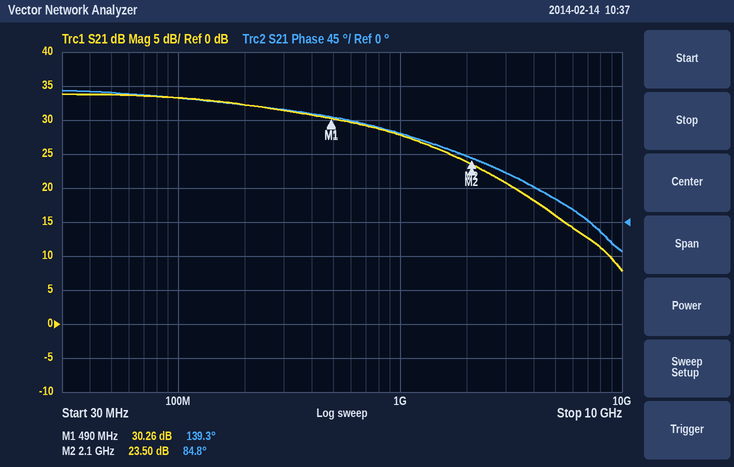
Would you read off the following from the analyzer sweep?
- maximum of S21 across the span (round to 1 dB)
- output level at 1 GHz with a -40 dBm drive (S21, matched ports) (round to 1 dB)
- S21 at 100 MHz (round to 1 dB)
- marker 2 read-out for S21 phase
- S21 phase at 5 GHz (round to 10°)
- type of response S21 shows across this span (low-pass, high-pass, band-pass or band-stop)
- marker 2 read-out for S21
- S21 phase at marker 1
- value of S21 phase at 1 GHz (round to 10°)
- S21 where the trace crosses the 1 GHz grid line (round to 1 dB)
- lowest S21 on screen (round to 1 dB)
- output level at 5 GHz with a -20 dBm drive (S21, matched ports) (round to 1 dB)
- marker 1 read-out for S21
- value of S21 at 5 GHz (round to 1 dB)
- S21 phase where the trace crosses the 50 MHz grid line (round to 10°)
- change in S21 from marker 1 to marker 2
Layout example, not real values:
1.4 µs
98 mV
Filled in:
34 dB
-12 dBm
33 dB
84.8°
30°
low-pass
23.50 dB
139.3°
120°
28 dB
8 dB
-4 dBm
30.26 dB
16 dB
170°
-6.76 dB
